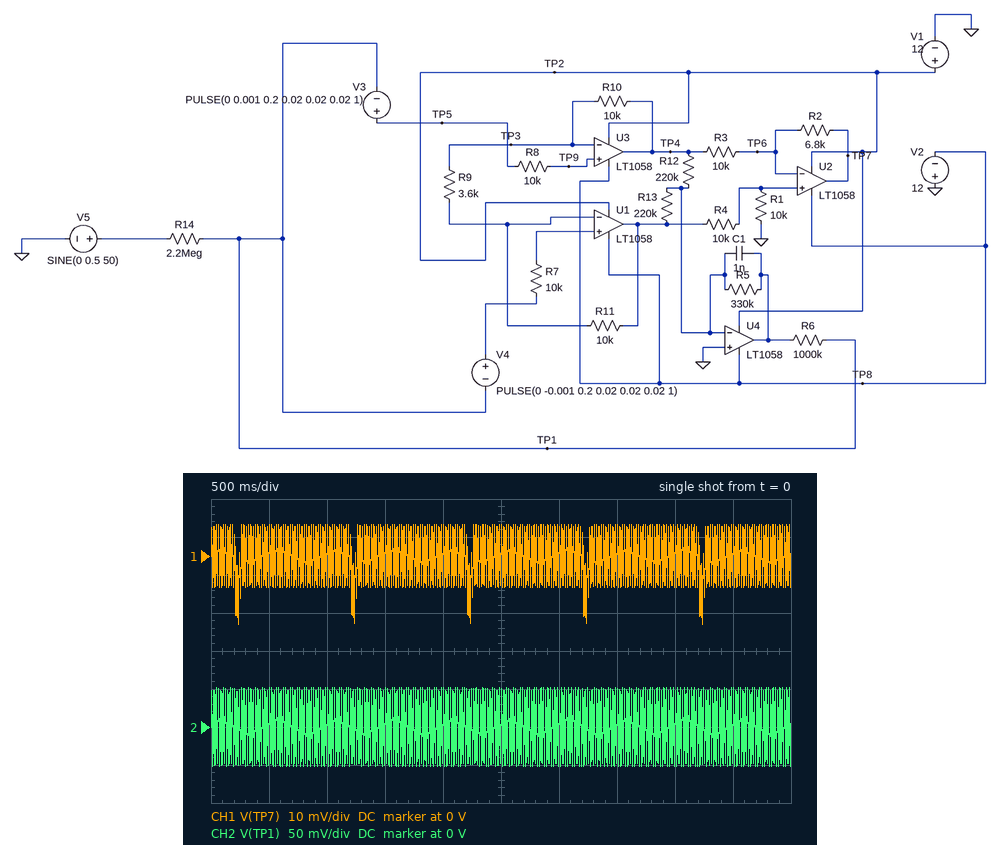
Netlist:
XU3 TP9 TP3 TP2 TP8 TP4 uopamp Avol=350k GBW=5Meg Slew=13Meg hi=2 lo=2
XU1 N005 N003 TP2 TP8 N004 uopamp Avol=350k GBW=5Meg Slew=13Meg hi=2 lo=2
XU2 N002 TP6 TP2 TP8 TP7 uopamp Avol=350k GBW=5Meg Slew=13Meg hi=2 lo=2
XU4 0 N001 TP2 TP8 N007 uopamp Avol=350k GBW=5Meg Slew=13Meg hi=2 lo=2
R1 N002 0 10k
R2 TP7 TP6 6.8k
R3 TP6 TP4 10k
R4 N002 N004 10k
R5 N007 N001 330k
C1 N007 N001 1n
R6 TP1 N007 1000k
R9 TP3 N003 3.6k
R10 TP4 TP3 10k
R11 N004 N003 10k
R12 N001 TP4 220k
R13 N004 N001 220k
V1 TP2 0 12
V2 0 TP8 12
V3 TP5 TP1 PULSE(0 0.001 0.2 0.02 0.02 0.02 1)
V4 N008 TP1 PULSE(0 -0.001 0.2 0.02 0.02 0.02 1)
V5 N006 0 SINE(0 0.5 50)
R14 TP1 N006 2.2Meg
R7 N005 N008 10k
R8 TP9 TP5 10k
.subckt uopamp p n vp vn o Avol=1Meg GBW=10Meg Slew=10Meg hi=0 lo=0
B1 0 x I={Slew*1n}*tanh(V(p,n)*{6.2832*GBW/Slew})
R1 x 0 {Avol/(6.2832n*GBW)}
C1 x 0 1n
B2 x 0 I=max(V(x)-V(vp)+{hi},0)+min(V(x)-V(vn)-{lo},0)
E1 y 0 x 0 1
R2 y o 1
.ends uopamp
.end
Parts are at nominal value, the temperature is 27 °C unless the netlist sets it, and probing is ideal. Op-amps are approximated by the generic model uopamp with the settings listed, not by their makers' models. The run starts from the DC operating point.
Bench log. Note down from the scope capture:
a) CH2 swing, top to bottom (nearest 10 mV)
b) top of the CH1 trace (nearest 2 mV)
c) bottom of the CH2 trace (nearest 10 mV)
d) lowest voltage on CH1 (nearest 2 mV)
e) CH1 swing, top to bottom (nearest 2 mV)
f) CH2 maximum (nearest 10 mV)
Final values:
100 mV
8 mV
-50 mV
-18 mV
26 mV
50 mV
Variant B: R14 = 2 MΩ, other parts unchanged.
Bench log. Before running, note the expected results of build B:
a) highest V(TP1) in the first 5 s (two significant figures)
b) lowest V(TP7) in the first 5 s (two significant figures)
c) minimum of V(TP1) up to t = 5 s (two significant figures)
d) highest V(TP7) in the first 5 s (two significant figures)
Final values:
56 mV
-19 mV
-56 mV
8.9 mV
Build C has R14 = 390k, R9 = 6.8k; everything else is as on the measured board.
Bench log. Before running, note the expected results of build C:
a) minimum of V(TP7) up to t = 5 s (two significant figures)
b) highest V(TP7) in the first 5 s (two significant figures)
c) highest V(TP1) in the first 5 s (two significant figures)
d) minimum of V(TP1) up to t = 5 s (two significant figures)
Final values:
-37 mV
31 mV
200 mV
-200 mV
